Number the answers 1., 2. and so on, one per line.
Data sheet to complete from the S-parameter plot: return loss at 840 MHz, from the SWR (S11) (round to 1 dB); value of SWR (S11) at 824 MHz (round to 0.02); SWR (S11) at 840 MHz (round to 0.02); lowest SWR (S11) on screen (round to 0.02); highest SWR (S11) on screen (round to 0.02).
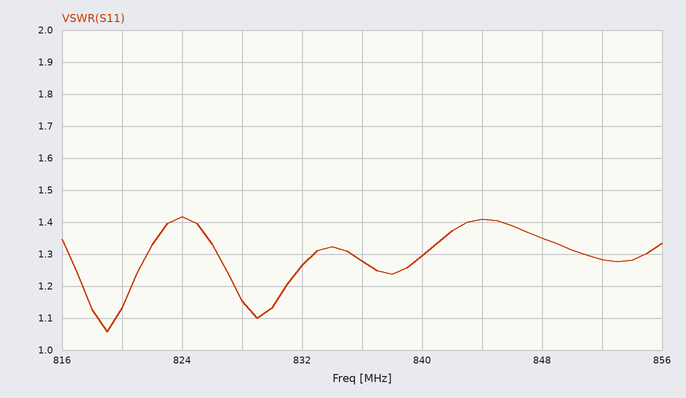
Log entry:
1. 18 dB
2. 1.42
3. 1.30
4. 1.06
5. 1.42
